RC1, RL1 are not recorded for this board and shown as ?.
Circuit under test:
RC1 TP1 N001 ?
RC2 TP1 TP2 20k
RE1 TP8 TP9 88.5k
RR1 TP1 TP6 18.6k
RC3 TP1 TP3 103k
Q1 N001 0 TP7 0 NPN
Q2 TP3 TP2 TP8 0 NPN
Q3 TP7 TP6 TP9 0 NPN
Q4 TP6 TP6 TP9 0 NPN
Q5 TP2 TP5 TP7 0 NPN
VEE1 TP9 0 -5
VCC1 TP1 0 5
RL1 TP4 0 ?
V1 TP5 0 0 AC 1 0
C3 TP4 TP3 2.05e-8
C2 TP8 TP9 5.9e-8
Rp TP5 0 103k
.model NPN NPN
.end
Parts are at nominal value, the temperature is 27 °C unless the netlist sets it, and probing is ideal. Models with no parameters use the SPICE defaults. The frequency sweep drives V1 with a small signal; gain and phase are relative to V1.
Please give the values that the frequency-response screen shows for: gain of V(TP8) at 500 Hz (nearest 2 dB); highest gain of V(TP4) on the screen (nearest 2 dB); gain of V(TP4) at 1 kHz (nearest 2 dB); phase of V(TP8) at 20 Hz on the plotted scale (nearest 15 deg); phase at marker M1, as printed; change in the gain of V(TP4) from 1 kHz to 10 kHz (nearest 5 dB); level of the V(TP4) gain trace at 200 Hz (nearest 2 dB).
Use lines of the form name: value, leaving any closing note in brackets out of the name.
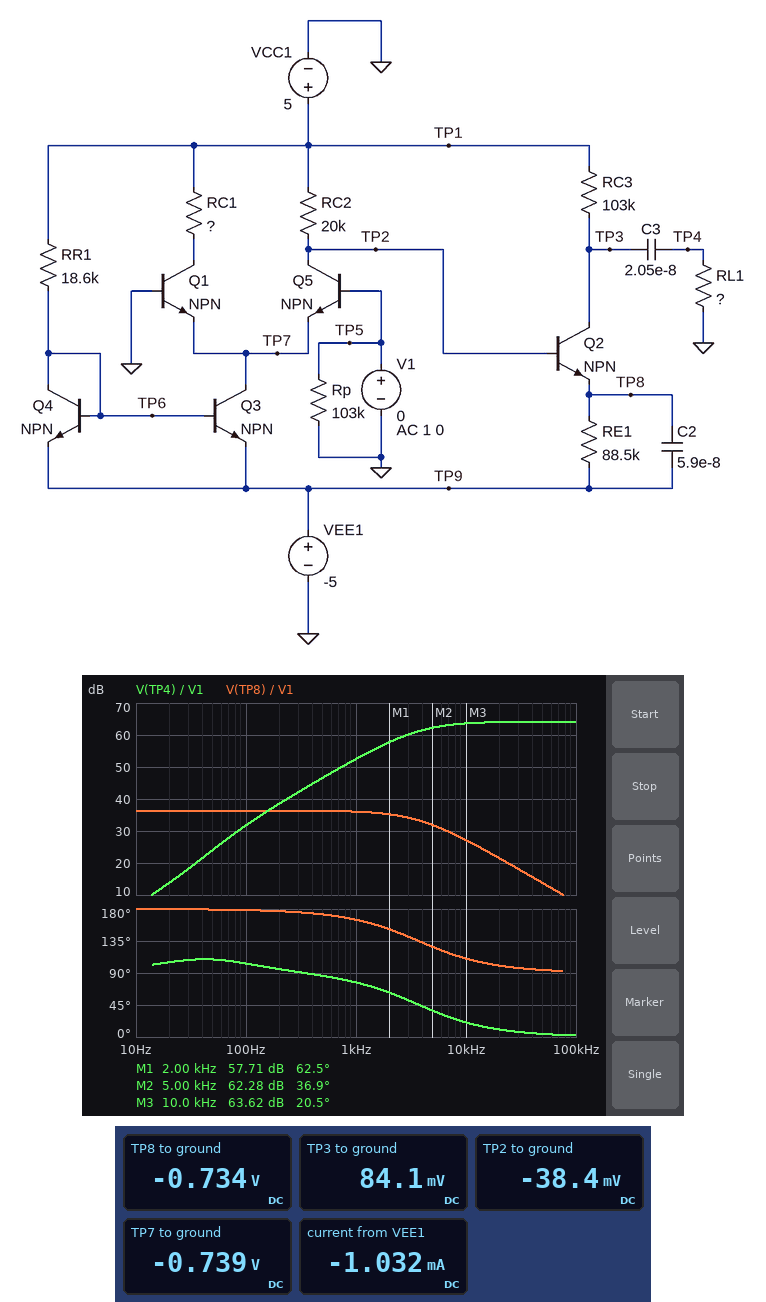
gain of V(TP8) at 500 Hz: 36 dB
highest gain of V(TP4) on the screen: 64 dB
gain of V(TP4) at 1 kHz: 52 dB
phase of V(TP8) at 20 Hz on the plotted scale: 180 deg
phase at marker M1, as printed: 62.5 deg
change in the gain of V(TP4) from 1 kHz to 10 kHz: 10 dB
level of the V(TP4) gain trace at 200 Hz: 38 dB
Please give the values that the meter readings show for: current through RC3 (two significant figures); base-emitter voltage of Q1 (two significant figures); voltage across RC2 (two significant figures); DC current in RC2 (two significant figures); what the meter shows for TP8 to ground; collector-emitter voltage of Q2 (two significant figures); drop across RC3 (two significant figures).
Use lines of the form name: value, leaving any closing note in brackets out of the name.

current through RC3: 48 µA
base-emitter voltage of Q1: 740 mV
voltage across RC2: 5.0 V
DC current in RC2: 250 µA
what the meter shows for TP8 to ground: -0.734 V
collector-emitter voltage of Q2: 820 mV
drop across RC3: 4.9 V
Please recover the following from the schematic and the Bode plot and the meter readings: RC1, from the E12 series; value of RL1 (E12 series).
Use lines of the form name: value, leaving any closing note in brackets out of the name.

RC1, from the E12 series: 27 kΩ
value of RL1: 22 kΩ
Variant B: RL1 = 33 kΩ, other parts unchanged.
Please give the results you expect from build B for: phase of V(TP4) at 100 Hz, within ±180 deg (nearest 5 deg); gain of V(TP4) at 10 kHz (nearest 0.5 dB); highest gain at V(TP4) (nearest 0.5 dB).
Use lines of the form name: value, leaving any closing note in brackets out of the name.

phase of V(TP4) at 100 Hz, within ±180 deg: 100 deg
gain of V(TP4) at 10 kHz: 66.5 dB
highest gain at V(TP4): 67.0 dB
